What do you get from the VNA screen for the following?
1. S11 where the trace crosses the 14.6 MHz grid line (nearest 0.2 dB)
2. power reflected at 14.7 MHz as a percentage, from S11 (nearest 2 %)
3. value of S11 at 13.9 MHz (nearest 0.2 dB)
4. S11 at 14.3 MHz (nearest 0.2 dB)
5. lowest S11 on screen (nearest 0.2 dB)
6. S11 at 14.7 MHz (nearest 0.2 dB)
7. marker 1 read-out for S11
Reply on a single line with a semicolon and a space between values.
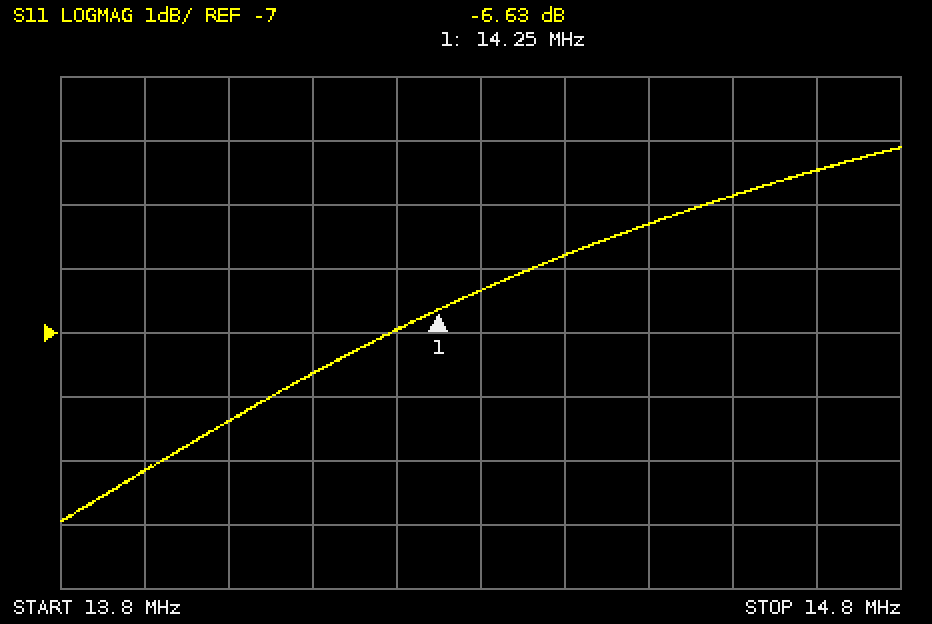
-4.8 dB; 36 %; -9.2 dB; -6.4 dB; -10.0 dB; -4.4 dB; -6.63 dB
